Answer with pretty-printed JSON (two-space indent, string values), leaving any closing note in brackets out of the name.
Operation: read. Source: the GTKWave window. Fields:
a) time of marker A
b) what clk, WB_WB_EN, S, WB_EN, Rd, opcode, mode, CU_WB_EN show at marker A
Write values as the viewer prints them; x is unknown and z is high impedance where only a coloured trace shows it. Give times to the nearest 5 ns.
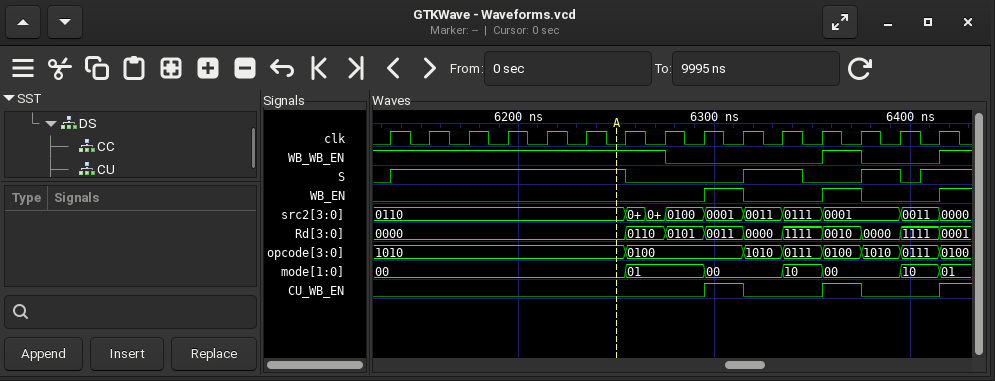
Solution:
{
  "time of marker A": "6250 ns",
  "what clk, WB_WB_EN, S, WB_EN, Rd, opcode, mode, CU_WB_EN show at marker A": "clk=0, WB_WB_EN=1, S=1, WB_EN=0, Rd=0000, opcode=1010, mode=00, CU_WB_EN=0"
}
